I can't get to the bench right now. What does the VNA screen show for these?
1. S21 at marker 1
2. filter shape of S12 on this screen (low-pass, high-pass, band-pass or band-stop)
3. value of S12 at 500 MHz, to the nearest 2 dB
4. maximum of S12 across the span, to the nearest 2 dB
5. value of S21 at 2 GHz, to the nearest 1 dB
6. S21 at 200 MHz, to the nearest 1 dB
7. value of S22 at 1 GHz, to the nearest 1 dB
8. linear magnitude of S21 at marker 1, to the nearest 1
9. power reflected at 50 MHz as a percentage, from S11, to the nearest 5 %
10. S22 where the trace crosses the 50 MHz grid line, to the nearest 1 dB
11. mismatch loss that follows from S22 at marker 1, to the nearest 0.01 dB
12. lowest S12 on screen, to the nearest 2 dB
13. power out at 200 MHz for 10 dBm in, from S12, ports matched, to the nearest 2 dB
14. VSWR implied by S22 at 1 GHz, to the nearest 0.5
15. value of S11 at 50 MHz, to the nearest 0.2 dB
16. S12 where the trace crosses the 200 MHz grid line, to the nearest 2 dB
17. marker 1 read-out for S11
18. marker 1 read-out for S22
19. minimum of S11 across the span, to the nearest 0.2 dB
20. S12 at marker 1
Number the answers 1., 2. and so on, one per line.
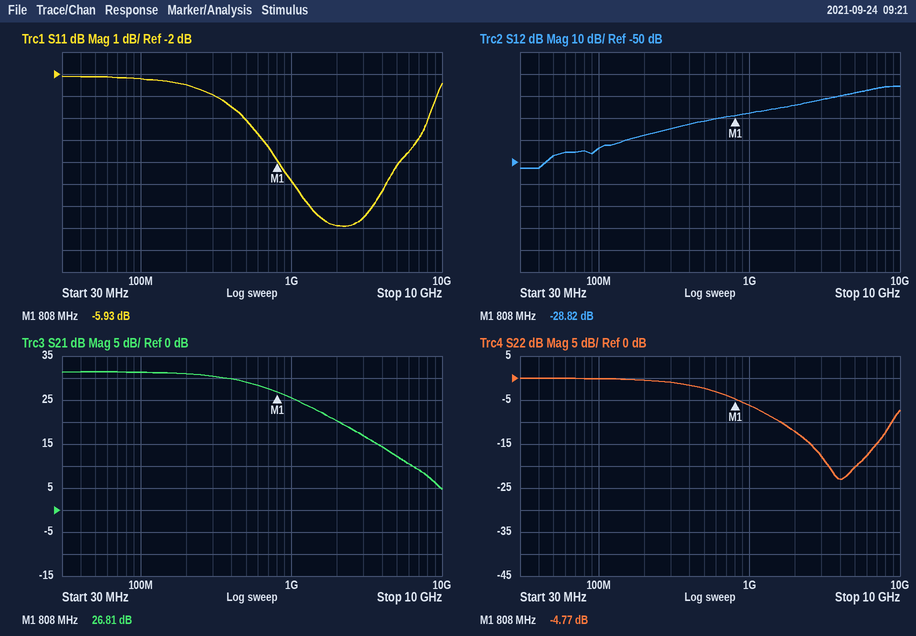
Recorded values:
1. 26.81 dB
2. high-pass
3. -32 dB
4. -16 dB
5. 20 dB
6. 31 dB
7. -6 dB
8. 22
9. 60 %
10. 0 dB
11. 1.76 dB
12. -52 dB
13. -28 dBm
14. 3.0
15. -2.2 dB
16. -38 dB
17. -5.93 dB
18. -4.77 dB
19. -9.0 dB
20. -28.82 dB
